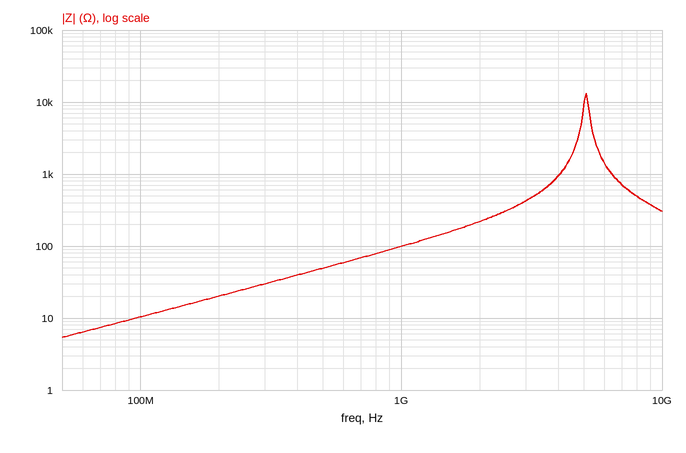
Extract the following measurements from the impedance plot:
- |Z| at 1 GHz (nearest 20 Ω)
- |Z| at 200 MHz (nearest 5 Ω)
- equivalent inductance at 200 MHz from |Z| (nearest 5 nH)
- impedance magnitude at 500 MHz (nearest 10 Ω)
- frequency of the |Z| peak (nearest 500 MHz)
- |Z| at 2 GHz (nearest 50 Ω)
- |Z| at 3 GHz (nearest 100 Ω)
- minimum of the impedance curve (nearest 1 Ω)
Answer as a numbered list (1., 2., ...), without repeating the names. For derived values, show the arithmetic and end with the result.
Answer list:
1. 100 Ω
2. 20 Ω
3. L = 20 Ω/(2π × 200 MHz) ≈ 15.9 nH, so 15 nH to the nearest 5 nH
4. 50 Ω
5. 5.0 GHz
6. 200 Ω
7. 400 Ω
8. 5 Ω
